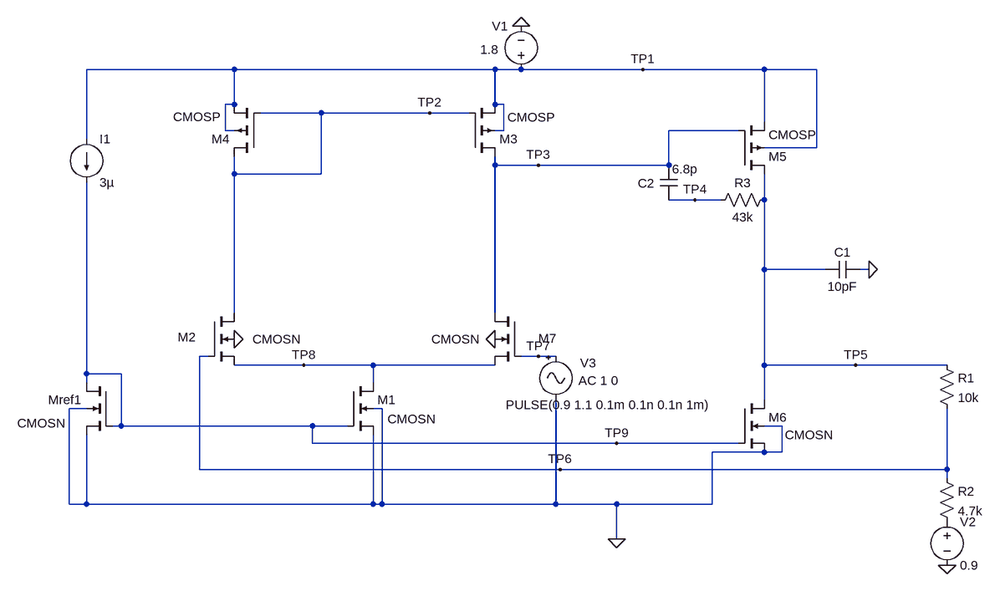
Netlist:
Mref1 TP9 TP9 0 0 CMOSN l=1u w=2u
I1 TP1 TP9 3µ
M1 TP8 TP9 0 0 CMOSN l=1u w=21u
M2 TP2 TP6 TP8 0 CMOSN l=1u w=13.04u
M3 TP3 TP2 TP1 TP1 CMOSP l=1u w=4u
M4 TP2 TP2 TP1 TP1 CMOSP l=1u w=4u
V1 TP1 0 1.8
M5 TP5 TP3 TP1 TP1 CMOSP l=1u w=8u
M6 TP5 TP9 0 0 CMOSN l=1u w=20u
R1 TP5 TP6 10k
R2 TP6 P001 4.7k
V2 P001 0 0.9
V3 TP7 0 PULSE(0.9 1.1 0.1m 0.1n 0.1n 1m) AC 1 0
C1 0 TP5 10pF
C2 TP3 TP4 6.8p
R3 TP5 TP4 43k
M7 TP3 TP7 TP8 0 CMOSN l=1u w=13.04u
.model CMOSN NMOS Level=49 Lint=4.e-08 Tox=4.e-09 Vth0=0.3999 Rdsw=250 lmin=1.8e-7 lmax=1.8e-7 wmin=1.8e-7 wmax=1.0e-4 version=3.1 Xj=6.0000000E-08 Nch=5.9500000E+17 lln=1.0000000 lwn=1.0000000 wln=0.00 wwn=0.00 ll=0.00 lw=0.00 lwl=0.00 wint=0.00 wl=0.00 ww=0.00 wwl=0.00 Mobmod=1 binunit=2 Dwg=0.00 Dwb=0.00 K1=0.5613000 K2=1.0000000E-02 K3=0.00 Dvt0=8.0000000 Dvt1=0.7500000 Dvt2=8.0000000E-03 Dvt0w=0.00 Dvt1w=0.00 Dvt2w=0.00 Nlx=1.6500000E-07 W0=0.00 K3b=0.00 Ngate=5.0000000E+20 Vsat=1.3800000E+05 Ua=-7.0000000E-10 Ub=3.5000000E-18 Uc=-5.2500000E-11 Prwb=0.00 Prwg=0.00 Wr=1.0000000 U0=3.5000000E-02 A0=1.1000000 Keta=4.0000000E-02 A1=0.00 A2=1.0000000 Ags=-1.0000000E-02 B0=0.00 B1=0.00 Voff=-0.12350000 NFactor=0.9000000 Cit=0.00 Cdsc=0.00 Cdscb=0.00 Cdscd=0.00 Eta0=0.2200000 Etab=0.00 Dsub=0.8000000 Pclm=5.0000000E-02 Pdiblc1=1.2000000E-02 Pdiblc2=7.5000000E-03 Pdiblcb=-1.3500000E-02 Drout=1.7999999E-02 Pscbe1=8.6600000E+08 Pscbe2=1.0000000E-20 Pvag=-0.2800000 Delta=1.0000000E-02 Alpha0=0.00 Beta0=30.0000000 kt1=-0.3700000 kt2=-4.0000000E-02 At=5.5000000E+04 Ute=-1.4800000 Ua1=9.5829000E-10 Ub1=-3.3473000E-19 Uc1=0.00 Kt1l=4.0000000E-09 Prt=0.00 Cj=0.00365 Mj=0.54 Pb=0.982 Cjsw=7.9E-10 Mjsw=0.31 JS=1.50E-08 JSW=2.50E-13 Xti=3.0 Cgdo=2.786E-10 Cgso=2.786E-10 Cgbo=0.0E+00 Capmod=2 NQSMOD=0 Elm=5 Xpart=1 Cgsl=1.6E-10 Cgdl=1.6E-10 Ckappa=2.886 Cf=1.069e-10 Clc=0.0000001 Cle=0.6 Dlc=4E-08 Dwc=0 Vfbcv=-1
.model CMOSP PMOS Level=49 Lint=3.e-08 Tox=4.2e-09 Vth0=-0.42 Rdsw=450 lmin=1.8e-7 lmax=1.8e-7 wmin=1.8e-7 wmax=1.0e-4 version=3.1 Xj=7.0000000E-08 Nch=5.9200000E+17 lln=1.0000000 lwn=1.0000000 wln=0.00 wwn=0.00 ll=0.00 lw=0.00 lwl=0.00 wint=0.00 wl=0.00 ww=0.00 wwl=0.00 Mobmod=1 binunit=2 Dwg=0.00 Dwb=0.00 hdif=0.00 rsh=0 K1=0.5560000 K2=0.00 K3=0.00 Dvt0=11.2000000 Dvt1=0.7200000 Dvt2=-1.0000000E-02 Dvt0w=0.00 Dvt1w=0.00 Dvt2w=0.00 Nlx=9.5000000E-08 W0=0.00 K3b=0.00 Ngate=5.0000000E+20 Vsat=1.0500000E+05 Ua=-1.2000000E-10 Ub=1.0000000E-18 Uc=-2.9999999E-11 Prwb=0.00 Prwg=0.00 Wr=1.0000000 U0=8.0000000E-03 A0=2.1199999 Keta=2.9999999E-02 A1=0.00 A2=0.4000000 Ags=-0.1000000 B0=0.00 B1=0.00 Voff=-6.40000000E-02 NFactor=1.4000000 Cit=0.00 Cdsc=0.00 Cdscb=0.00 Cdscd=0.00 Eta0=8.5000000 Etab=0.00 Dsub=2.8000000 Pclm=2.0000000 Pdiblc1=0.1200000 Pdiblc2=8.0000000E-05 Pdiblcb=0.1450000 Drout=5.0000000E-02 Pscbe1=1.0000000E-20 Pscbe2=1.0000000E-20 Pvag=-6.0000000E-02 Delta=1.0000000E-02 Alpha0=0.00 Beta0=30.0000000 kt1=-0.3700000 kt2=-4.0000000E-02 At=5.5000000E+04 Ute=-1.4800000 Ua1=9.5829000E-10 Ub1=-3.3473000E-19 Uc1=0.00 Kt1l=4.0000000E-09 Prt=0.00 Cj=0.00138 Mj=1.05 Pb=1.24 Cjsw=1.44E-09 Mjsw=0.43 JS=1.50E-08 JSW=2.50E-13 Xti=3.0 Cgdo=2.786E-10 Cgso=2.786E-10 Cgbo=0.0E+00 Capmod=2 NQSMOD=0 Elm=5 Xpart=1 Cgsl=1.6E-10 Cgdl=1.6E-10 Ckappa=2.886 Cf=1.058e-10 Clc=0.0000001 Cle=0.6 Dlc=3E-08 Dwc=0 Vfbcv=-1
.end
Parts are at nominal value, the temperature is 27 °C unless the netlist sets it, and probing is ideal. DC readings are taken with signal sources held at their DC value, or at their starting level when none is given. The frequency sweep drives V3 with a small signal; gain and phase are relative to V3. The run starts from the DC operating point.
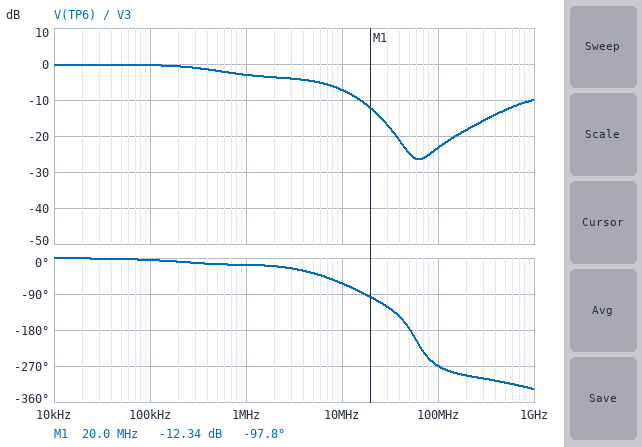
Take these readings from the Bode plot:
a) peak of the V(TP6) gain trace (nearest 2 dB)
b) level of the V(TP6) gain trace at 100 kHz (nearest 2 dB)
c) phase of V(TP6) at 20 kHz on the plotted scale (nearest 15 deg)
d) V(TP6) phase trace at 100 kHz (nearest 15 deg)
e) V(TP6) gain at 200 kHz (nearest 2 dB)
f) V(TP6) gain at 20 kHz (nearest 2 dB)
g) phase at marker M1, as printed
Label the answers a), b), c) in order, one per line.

a) 0 dB
b) 0 dB
c) 0 deg
d) 0 deg
e) 0 dB
f) 0 dB
g) -97.8 deg
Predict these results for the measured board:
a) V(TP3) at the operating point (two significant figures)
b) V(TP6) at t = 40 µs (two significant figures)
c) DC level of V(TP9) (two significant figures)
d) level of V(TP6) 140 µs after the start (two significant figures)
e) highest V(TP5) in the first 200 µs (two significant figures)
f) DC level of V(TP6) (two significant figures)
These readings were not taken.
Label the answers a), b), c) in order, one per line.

a) 950 mV
b) 900 mV
c) 520 mV
d) 1.1 V
e) 1.5 V
f) 900 mV
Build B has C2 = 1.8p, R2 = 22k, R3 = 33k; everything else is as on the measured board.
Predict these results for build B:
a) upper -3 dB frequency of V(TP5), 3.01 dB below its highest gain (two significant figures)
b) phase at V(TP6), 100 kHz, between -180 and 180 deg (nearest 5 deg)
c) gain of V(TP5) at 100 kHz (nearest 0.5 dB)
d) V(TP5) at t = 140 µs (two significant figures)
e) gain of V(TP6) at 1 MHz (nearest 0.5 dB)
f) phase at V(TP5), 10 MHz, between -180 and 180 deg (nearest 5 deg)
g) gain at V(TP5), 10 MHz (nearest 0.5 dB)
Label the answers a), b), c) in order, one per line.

a) 11 MHz
b) 0 deg
c) 3.0 dB
d) 1.2 V
e) 0 dB
f) -60 deg
g) 0.5 dB
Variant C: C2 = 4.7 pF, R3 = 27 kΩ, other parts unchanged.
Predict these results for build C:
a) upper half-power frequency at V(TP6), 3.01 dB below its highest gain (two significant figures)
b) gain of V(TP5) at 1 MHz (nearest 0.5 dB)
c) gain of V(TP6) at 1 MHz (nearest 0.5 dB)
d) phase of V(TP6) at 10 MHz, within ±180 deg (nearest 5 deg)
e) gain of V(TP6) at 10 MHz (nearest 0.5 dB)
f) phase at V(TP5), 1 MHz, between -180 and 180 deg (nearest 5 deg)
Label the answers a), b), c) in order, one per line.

a) 1.5 MHz
b) 7.5 dB
c) -2.0 dB
d) -75 deg
e) -11.5 dB
f) -25 deg
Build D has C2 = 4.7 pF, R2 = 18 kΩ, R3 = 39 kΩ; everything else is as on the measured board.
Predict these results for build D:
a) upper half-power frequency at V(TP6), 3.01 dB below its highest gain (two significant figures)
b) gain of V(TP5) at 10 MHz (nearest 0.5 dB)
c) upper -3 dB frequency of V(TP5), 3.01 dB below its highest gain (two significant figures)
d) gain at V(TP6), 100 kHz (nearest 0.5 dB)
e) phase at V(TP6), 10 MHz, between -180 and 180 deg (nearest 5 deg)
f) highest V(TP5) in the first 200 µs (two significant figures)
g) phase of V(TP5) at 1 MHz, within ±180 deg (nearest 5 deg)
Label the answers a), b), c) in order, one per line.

a) 9.3 MHz
b) 0.5 dB
c) 9.7 MHz
d) 0 dB
e) -50 deg
f) 1.2 V
g) -10 deg
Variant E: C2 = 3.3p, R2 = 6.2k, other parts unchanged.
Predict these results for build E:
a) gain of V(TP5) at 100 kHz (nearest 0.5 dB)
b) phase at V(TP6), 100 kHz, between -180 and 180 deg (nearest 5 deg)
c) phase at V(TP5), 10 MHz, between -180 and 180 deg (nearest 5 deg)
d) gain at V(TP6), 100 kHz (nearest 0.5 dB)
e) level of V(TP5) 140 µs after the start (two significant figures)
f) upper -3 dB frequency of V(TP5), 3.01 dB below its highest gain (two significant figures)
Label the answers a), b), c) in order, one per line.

a) 8.0 dB
b) 0 deg
c) -60 deg
d) 0 dB
e) 1.4 V
f) 4.3 MHz
